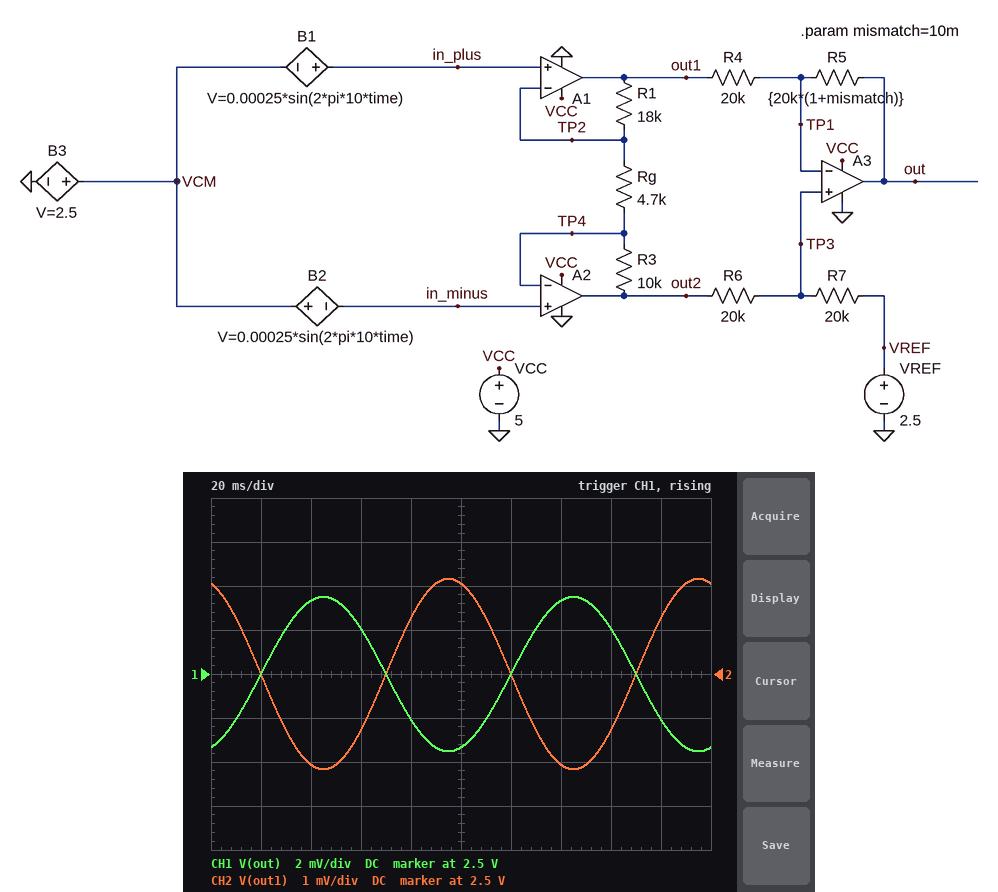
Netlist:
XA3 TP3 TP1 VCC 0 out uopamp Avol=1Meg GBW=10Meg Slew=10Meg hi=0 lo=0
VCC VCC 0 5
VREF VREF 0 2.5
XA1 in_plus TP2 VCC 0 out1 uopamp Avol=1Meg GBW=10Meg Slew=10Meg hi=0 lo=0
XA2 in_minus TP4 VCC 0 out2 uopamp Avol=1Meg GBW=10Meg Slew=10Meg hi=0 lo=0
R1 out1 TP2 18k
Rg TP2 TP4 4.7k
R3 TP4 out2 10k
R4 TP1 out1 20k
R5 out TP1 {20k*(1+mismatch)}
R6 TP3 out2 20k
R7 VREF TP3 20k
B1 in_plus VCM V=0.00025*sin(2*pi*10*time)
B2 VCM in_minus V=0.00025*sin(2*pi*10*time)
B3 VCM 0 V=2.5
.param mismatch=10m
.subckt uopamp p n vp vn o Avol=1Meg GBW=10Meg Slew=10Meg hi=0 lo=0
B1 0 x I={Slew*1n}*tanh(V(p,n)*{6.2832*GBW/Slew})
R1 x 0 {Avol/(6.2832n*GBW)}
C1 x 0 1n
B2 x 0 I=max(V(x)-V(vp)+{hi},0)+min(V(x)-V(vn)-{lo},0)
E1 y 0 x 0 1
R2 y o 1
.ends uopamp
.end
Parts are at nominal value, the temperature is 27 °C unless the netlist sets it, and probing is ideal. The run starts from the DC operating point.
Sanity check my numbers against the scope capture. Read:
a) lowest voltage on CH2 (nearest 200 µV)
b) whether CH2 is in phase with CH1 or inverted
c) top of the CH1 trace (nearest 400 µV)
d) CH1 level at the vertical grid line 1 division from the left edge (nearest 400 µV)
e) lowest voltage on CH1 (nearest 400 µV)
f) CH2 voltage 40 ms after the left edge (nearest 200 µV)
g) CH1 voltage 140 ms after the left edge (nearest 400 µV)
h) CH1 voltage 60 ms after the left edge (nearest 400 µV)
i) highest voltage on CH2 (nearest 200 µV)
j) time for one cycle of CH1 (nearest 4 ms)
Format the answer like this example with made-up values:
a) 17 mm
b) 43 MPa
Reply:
a) 2.4978 V
b) inverted
c) 2.5036 V
d) 2.5000 V
e) 2.4964 V
f) 2.4980 V
g) 2.5032 V
h) 2.5020 V
i) 2.5022 V
j) 100 ms
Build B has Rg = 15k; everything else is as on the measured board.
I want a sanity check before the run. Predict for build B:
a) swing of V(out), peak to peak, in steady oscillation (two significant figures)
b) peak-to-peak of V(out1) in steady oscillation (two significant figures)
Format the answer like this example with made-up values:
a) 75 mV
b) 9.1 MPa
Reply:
a) 2.9 mV
b) 1.7 mV
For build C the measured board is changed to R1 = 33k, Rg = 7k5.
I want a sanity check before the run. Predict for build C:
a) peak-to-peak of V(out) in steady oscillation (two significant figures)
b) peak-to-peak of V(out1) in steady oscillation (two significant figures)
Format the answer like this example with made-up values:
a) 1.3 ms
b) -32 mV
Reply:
a) 6.8 mV
b) 4.9 mV
